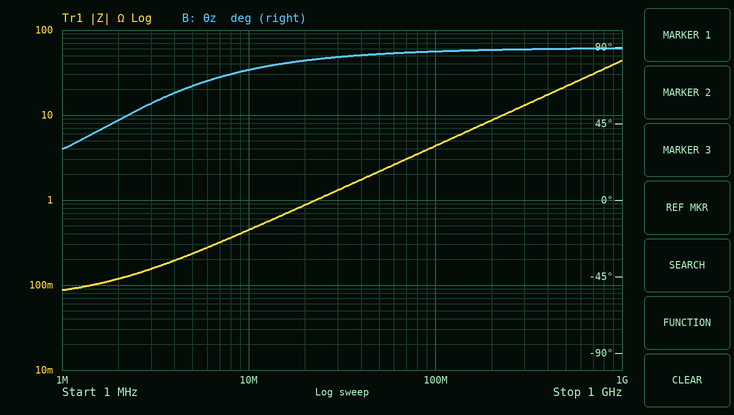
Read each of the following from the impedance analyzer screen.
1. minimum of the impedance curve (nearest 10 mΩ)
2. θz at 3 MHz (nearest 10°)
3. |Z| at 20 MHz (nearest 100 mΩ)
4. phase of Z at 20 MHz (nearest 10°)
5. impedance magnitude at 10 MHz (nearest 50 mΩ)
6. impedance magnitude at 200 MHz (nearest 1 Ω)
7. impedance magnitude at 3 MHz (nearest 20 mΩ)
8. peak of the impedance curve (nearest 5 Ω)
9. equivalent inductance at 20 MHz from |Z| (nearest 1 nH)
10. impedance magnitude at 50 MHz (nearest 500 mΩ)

90 mΩ
60°
900 mΩ
80°
450 mΩ
9 Ω
160 mΩ
45 Ω
7 nH
2.0 Ω
